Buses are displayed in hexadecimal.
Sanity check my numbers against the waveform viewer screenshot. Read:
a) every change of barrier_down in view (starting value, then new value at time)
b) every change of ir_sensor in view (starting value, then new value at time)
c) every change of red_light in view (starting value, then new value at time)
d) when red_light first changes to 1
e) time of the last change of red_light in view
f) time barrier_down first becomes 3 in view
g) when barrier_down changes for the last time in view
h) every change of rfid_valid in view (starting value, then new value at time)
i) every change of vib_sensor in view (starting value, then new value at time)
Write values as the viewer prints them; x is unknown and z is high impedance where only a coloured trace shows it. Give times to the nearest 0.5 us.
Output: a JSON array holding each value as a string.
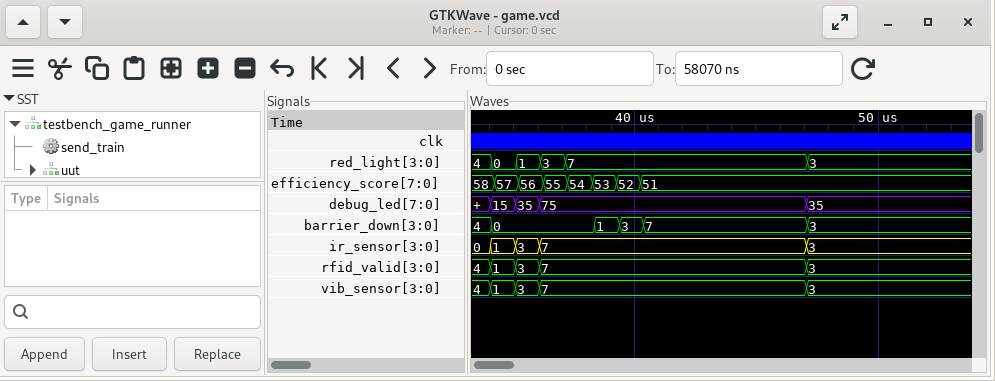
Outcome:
["4, 0 at 34 us, 1 at 38.5 us, 3 at 39.5 us, 7 at 40.5 us, 3 at 47 us", "0, 1 at 34 us, 3 at 35 us, 7 at 36 us, 3 at 47 us", "4, 0 at 34 us, 1 at 35 us, 3 at 36 us, 7 at 37 us, 3 at 47 us", "35 us", "47 us", "39.5 us", "47 us", "4, 1 at 34 us, 3 at 35 us, 7 at 36 us, 3 at 47 us", "4, 1 at 34 us, 3 at 35 us, 7 at 36 us, 3 at 47 us"]
